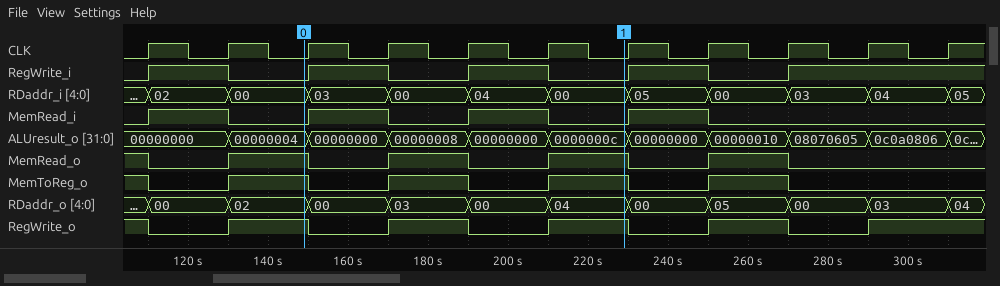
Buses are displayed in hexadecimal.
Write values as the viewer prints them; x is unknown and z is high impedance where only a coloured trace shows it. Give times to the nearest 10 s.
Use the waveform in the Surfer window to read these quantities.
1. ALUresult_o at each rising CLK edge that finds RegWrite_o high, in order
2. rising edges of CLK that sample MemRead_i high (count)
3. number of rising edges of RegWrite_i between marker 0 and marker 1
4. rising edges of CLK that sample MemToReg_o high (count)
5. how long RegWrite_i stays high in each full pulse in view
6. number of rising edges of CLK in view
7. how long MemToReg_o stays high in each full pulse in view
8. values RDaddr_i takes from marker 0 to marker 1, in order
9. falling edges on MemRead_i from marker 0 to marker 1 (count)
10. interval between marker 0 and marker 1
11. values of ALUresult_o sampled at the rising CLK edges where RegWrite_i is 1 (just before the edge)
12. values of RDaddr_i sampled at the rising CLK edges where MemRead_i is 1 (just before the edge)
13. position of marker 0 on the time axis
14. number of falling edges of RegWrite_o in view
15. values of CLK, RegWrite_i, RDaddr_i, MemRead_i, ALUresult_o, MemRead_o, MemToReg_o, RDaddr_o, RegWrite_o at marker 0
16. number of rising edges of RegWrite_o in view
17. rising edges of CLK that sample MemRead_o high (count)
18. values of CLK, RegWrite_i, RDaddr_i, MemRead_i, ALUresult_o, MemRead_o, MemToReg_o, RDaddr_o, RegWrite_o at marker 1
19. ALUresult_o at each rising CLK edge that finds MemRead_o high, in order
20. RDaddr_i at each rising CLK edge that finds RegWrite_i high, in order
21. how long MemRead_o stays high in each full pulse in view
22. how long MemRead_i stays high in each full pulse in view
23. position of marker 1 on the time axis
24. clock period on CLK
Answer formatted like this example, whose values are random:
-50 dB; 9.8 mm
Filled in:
00000000, 00000004, 00000008, 0000000c, 00000010, 0c0a0806; 4; 2; 5; 20 s, 20 s, 20 s, 20 s; 11; 20 s, 20 s, 20 s, 20 s; 00, 03, 00, 04, 00; 2; 80 s; 00000000, 00000000, 00000000, 00000000, 08070605, 0c0a0806; 02, 03, 04, 05; 150 s; 5; CLK=0, RegWrite_i=0, RDaddr_i=00, MemRead_i=0, ALUresult_o=00000004, MemRead_o=1, MemToReg_o=1, RDaddr_o=02, RegWrite_o=1; 5; 5; CLK=0, RegWrite_i=0, RDaddr_i=00, MemRead_i=0, ALUresult_o=0000000c, MemRead_o=1, MemToReg_o=1, RDaddr_o=04, RegWrite_o=1; 00000000, 00000004, 00000008, 0000000c, 00000010; 02, 03, 04, 05, 03, 04; 20 s, 20 s, 20 s, 20 s; 20 s, 20 s, 20 s, 20 s; 230 s; 20 s
